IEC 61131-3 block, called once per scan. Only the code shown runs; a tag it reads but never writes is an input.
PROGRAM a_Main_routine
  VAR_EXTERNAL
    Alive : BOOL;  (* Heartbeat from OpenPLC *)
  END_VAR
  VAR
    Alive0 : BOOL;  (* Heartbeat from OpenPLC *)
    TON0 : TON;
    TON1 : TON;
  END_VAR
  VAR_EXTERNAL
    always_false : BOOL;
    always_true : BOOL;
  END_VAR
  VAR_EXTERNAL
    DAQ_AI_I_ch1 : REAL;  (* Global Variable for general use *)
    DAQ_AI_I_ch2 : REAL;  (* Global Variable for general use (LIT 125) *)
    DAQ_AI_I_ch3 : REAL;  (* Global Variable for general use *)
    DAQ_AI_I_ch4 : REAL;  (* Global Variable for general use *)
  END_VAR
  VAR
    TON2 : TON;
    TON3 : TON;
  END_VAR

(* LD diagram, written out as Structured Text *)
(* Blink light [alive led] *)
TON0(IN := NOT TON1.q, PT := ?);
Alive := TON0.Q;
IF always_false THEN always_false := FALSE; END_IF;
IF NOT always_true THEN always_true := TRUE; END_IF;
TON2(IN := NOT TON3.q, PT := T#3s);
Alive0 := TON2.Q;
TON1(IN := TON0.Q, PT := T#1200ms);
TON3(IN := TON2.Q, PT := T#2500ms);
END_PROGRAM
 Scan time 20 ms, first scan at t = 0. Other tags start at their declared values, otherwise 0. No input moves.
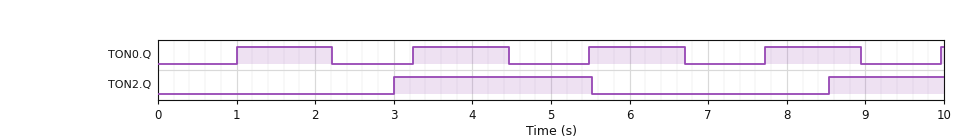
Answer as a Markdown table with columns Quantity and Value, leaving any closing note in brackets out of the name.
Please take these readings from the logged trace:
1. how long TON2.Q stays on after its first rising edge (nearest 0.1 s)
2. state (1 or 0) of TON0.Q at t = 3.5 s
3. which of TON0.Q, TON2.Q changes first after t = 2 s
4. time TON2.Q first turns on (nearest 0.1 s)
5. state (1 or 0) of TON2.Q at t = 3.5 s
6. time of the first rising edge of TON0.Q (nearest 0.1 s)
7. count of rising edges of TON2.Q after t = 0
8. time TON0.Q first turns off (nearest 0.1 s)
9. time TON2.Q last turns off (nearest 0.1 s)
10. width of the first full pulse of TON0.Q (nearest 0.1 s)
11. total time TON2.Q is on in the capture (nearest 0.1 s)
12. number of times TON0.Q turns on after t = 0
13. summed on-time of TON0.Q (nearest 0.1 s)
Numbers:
| Quantity | Value |
|---|---|
| how long TON2.Q stays on after its first rising edge | 2.5 s |
| state (1 or 0) of TON0.Q at t = 3.5 s | 1 |
| which of TON0.Q, TON2.Q changes first after t = 2 s | TON0.Q |
| time TON2.Q first turns on | 3.0 s |
| state (1 or 0) of TON2.Q at t = 3.5 s | 1 |
| time of the first rising edge of TON0.Q | 1.0 s |
| count of rising edges of TON2.Q after t = 0 | 2 |
| time TON0.Q first turns off | 2.2 s |
| time TON2.Q last turns off | 5.5 s |
| width of the first full pulse of TON0.Q | 1.2 s |
| total time TON2.Q is on in the capture | 4.0 s |
| number of times TON0.Q turns on after t = 0 | 5 |
| summed on-time of TON0.Q | 4.9 s |
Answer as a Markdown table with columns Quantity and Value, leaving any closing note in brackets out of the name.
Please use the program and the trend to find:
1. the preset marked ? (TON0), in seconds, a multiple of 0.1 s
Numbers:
| Quantity | Value |
|---|---|
| the preset marked ? (TON0), in seconds, a multiple of 0.1 s | 1.0 s |
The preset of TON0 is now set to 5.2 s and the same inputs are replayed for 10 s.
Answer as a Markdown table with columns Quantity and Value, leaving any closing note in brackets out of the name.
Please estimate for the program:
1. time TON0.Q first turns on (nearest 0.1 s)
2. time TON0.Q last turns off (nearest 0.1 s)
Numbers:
| Quantity | Value |
|---|---|
| time TON0.Q first turns on | 5.2 s |
| time TON0.Q last turns off | 6.4 s |
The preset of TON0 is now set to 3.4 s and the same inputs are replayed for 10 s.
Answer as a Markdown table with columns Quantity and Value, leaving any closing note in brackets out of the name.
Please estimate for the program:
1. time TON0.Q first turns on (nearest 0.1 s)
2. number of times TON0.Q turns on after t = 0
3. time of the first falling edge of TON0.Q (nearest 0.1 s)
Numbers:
| Quantity | Value |
|---|---|
| time TON0.Q first turns on | 3.4 s |
| number of times TON0.Q turns on after t = 0 | 2 |
| time of the first falling edge of TON0.Q | 4.6 s |
